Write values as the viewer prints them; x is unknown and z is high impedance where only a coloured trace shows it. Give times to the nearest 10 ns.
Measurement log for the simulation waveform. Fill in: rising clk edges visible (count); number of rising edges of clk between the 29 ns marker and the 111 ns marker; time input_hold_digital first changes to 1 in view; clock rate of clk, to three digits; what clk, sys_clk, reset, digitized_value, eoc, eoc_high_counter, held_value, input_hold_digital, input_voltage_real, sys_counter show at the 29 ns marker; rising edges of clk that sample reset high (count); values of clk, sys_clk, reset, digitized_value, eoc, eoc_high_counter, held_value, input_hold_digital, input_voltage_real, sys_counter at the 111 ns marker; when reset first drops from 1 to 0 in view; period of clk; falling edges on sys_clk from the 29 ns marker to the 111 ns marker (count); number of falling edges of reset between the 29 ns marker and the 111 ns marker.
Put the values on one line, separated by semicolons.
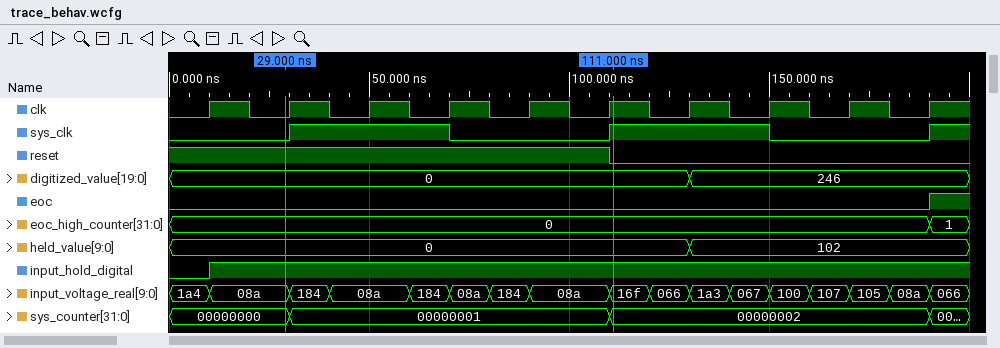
10; 5; 10 ns; 50.0 MHz; clk=0, sys_clk=0, reset=1, digitized_value=0, eoc=0, eoc_high_counter=0, held_value=0, input_hold_digital=1, input_voltage_real=08a, sys_counter=00000000; 6; clk=1, sys_clk=1, reset=0, digitized_value=0, eoc=0, eoc_high_counter=0, held_value=0, input_hold_digital=1, input_voltage_real=16f, sys_counter=00000002; 110 ns; 20 ns; 1; 1
